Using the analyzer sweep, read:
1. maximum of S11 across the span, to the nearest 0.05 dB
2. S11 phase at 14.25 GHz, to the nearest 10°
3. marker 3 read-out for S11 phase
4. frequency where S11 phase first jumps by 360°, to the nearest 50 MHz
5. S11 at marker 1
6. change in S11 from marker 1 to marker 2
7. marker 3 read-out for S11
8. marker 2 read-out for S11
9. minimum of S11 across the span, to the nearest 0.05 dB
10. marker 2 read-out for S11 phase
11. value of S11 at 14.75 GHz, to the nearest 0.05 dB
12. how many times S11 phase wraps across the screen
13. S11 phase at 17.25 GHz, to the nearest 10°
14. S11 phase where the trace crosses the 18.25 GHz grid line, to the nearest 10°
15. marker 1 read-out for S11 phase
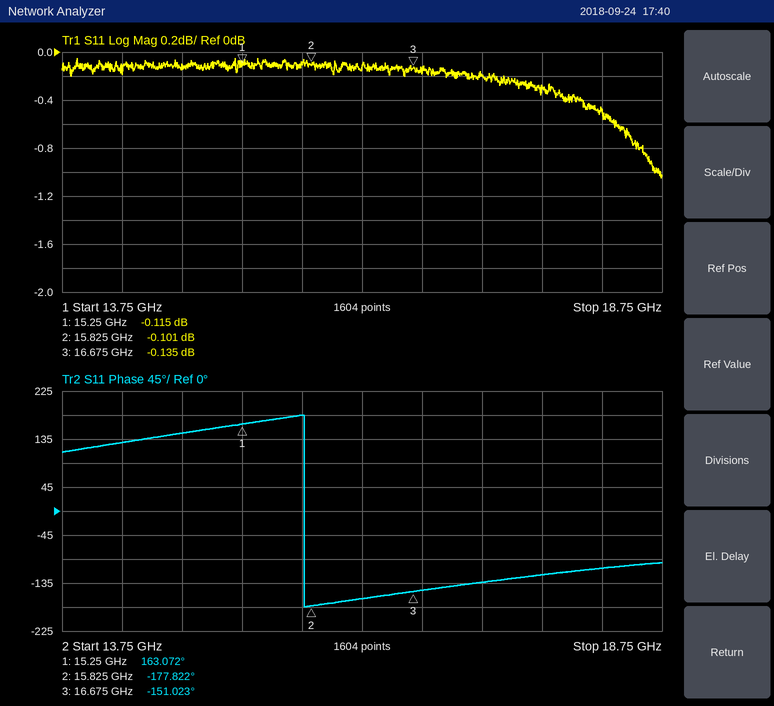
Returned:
-0.05 dB
130°
-151.023°
15.75 GHz
-0.115 dB
0.014 dB
-0.135 dB
-0.101 dB
-1.05 dB
-177.822°
-0.10 dB
1
-130°
-110°
163.072°
